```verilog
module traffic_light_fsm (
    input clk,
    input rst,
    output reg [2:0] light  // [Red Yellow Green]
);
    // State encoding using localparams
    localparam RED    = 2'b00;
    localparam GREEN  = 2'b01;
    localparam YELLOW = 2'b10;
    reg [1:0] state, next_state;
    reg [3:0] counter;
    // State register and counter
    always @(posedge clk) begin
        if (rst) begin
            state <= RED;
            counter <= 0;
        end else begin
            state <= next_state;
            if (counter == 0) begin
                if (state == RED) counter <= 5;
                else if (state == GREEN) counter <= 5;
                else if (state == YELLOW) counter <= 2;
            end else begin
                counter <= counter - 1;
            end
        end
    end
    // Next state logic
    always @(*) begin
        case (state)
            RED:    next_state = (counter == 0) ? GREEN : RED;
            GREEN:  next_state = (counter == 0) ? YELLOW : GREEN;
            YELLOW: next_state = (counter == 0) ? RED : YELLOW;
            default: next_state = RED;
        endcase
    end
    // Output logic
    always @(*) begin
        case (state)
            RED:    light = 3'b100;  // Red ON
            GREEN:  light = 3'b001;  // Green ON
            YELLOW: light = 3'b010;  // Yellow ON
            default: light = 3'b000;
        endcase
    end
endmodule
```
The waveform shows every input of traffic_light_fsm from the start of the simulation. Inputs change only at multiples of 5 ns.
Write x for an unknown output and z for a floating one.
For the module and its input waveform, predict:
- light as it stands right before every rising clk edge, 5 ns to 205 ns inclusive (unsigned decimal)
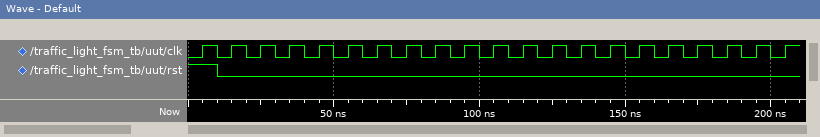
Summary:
x, 4, 1, 1, 1, 1, 1, 1, 2, 2, 2, 2, 2, 2, 4, 4, 4, 1, 1, 1, 1
